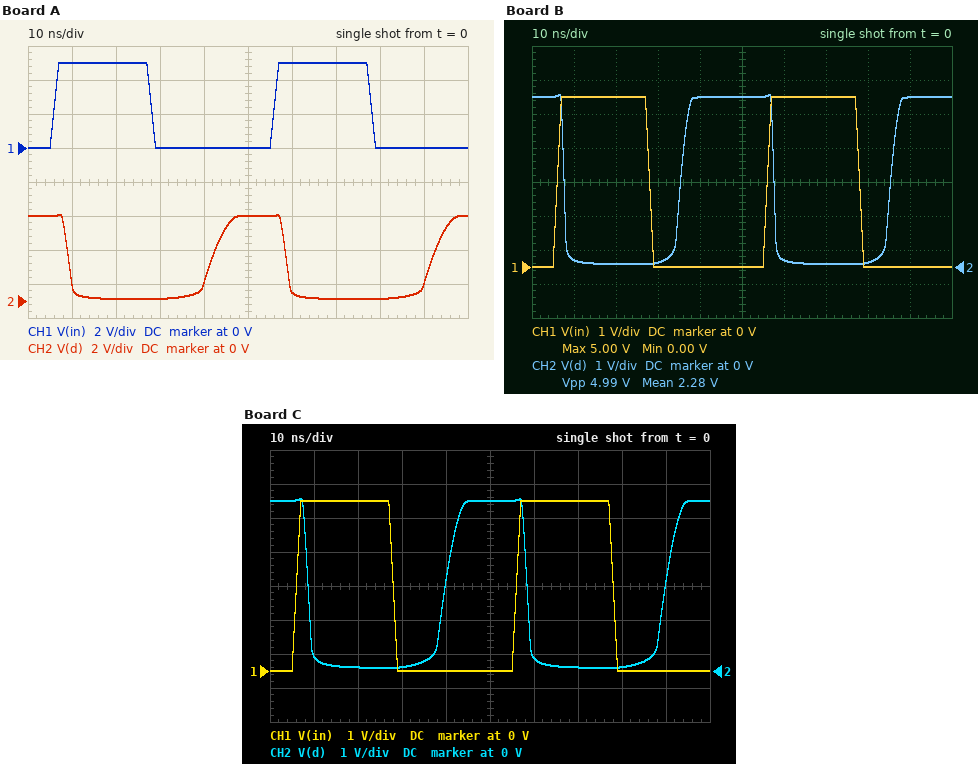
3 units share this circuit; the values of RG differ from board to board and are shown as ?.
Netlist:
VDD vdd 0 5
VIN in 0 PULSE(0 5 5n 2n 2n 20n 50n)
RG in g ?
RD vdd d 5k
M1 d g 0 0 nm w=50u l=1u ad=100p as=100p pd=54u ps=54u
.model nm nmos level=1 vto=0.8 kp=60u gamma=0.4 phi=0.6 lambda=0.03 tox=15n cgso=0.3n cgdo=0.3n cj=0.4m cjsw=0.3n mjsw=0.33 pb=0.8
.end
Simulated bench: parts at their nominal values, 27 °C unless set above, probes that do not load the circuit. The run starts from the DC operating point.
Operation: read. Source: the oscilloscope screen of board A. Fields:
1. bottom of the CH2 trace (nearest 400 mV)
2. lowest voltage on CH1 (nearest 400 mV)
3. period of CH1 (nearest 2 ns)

0 V
0 V
50 ns
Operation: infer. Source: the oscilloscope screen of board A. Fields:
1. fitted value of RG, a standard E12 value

68 kΩ
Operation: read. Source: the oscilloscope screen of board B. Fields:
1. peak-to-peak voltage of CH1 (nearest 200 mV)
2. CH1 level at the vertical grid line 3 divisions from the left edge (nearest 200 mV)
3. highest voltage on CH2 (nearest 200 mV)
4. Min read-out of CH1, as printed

5.0 V
0 V
5.0 V
0.00 V
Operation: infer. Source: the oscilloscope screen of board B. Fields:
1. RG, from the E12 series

33 kΩ
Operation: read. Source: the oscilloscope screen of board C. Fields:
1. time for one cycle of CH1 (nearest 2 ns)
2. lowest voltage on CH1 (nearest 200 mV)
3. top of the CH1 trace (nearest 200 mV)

50 ns
0 V
5.0 V
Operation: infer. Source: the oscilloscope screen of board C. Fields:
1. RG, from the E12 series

56 kΩ
